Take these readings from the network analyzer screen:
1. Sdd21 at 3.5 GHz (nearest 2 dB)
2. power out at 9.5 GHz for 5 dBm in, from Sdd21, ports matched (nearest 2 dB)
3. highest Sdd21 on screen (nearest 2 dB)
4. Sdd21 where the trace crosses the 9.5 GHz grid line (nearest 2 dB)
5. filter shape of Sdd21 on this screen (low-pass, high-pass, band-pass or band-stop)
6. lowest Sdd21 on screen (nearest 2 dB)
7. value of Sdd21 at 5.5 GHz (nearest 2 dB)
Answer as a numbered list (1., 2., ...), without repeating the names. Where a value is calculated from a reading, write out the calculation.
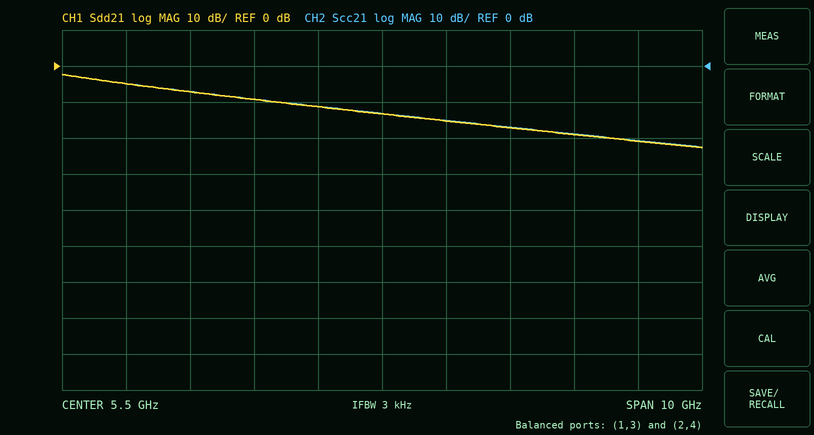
1. -10 dB
2. 5 dBm + (-20 dB) = -16 dBm
3. -2 dB
4. -20 dB
5. low-pass
6. -22 dB
7. -14 dB
